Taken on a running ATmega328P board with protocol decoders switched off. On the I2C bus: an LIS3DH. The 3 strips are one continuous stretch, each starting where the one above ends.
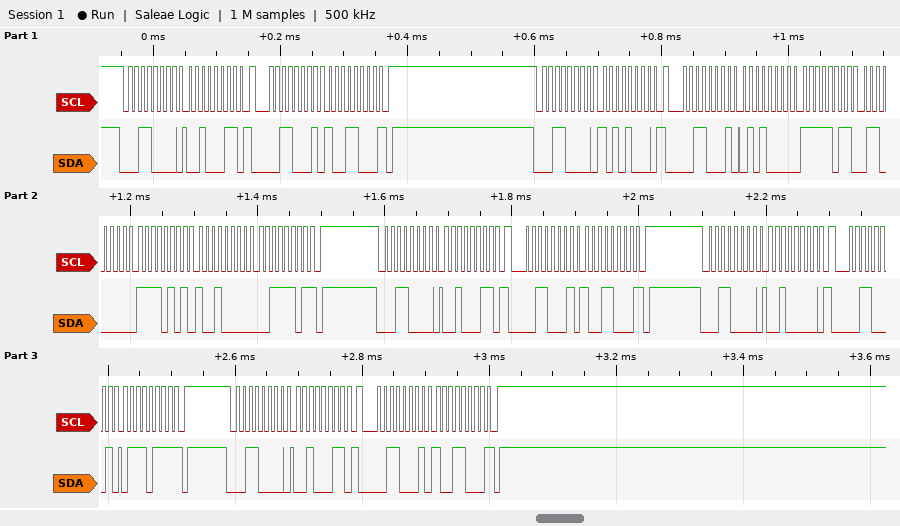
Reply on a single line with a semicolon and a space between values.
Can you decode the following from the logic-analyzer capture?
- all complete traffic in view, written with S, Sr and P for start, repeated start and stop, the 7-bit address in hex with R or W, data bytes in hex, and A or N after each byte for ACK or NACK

S 18W A 23 A Sr 18R A 98 N P S 18W A A8 A Sr 18R A 50 A FB A 60 A F5 A 90 A 3D N P S 18W A 23 A Sr 18R A 98 N P S 18W A 20 A Sr 18R A 77 N P S 18W A 23 A Sr 18R A 98 N P
